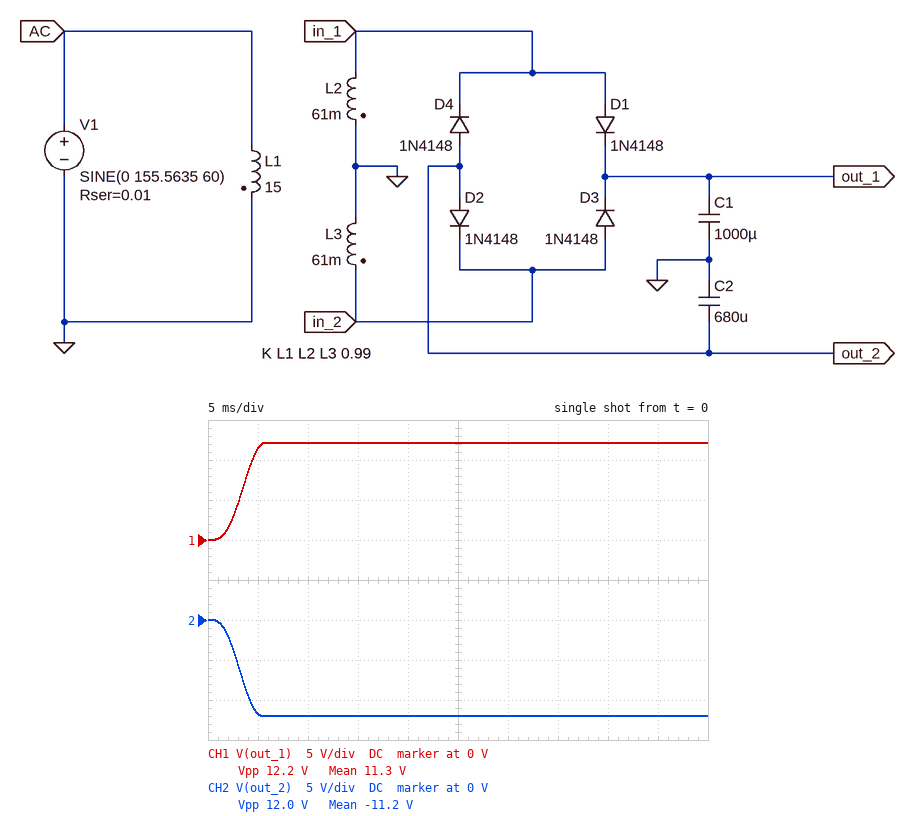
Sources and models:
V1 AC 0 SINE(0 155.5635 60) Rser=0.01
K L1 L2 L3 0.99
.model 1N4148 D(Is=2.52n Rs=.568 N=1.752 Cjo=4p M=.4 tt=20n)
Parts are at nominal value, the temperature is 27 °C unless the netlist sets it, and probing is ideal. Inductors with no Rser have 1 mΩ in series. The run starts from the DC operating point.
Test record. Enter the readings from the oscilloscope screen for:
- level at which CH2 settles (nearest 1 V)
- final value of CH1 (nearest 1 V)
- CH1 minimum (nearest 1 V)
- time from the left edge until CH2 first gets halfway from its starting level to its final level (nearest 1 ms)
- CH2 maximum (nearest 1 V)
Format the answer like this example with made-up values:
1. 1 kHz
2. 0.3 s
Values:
1. -12 V
2. 12 V
3. 0 V
4. 3 ms
5. 0 V
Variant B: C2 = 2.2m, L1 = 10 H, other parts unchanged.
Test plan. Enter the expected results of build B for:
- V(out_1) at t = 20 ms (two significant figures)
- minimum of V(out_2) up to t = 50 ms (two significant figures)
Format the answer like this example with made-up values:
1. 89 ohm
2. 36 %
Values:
1. 14 V
2. -13 V
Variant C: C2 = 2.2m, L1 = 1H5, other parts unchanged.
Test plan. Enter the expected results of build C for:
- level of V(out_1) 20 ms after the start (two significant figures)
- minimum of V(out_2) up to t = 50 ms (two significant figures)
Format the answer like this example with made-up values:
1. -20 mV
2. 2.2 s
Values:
1. 38 V
2. -36 V
